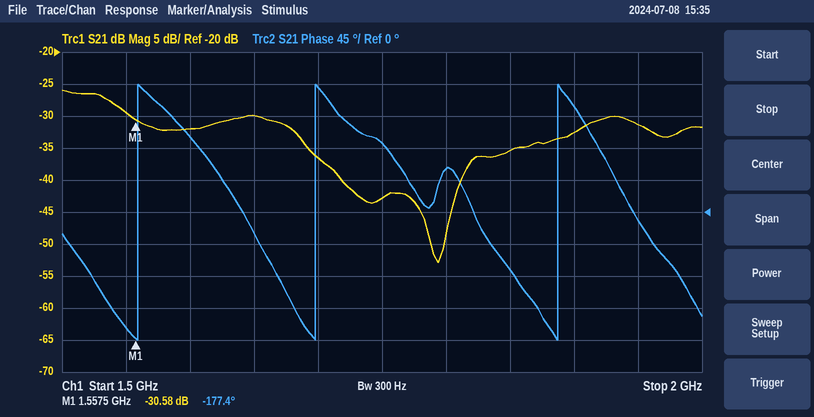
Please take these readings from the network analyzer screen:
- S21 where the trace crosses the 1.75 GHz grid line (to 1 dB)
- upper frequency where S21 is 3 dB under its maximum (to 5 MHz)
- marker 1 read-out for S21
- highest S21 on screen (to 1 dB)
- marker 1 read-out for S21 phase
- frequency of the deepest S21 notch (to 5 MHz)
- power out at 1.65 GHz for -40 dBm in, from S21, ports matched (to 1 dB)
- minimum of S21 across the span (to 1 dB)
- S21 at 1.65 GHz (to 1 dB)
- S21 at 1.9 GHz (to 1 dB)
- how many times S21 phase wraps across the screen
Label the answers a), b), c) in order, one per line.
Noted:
a) -43 dB
b) 1.545 GHz
c) -30.58 dB
d) -26 dB
e) -177.4°
f) 1.795 GHz
g) -70 dBm
h) -53 dB
i) -30 dB
j) -33 dB
k) 3
